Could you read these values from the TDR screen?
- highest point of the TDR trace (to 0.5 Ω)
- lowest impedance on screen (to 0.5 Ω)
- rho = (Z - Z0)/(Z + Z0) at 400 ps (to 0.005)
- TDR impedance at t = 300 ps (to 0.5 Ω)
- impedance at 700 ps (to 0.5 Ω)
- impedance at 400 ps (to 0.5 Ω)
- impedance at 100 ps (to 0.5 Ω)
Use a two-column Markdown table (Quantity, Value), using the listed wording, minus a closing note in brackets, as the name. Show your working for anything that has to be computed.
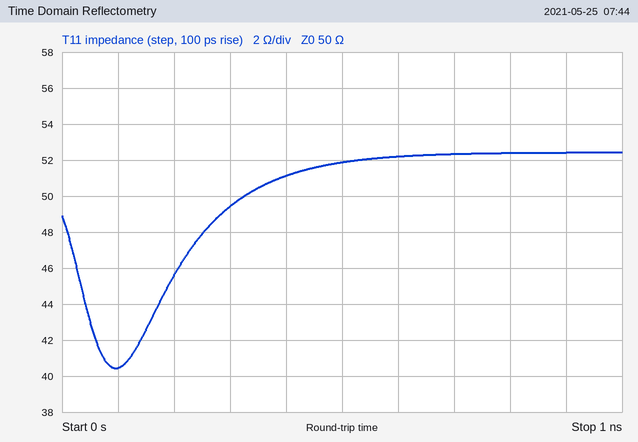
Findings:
| Quantity | Value |
|---|---|
| highest point of the TDR trace | 52.5 Ω |
| lowest impedance on screen | 40.5 Ω |
| rho = (Z - Z0)/(Z + Z0) at 400 ps | (51 − 50)/(51 + 50) ≈ +0.010 |
| TDR impedance at t = 300 ps | 49.5 Ω |
| impedance at 700 ps | 52.5 Ω |
| impedance at 400 ps | 51.0 Ω |
| impedance at 100 ps | 40.5 Ω |
